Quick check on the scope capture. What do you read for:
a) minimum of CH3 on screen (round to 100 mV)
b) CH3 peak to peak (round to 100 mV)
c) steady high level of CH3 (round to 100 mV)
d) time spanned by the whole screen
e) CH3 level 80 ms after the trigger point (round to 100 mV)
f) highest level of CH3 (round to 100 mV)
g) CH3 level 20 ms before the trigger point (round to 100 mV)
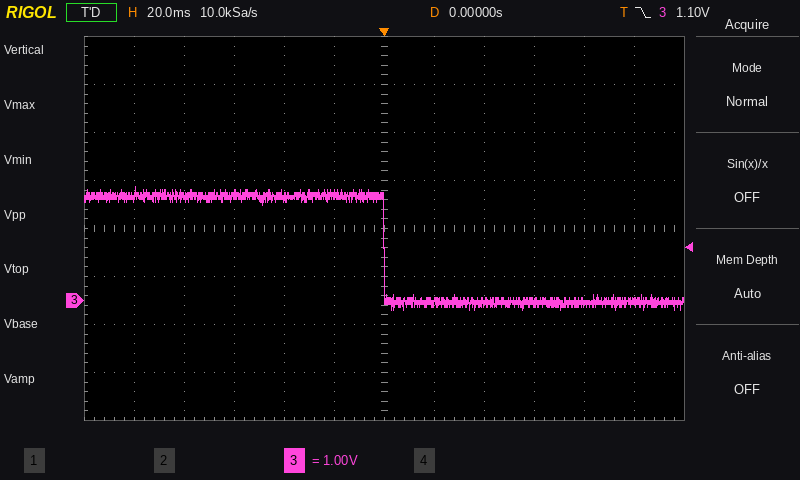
-200 mV
2.6 V
2.2 V
240 ms
0.0 V
2.4 V
2.2 V
